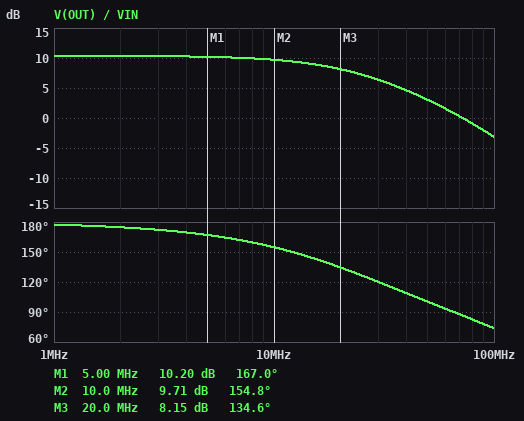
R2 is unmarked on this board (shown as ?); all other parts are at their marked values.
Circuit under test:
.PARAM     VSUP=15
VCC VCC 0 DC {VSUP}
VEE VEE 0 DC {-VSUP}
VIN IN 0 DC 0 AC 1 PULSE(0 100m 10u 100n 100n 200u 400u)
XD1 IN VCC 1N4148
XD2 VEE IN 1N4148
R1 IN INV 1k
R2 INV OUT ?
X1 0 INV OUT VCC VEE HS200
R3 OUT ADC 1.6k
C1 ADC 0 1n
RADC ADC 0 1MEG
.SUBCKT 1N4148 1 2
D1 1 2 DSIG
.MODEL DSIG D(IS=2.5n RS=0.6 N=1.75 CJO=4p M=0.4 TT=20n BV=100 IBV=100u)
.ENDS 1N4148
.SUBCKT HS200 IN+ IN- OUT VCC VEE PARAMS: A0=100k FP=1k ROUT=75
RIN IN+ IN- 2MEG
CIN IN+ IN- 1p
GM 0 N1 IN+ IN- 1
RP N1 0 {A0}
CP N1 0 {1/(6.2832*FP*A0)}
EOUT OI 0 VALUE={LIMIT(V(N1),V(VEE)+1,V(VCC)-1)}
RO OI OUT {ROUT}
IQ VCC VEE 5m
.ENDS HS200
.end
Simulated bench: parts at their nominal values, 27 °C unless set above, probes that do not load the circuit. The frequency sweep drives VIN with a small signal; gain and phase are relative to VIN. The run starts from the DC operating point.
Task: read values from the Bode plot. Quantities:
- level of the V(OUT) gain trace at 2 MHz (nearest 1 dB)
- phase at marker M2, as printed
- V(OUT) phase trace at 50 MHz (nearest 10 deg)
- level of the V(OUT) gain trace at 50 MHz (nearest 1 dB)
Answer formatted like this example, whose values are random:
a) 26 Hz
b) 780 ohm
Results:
a) 10 dB
b) 154.8 deg
c) 100 deg
d) 3 dB
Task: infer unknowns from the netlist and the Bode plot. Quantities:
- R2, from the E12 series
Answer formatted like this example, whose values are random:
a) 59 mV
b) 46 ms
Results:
a) 3.3 kΩ
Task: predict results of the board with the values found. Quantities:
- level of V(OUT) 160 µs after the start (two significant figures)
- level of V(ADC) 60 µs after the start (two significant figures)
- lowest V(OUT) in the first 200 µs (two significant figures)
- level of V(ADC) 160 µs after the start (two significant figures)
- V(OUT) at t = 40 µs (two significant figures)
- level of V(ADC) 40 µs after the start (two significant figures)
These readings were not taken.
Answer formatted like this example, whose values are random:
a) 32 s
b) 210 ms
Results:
a) -330 mV
b) -330 mV
c) -330 mV
d) -330 mV
e) -330 mV
f) -330 mV
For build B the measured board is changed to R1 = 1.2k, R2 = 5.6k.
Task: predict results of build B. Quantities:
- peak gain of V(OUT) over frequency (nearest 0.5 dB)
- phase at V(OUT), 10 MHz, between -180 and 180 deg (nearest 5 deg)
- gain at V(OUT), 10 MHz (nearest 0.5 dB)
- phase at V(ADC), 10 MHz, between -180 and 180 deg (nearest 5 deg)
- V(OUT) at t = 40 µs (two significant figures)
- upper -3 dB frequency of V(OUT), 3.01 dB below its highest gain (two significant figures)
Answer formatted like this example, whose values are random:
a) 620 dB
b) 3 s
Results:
a) 13.5 dB
b) 150 deg
c) 12.5 dB
d) 60 deg
e) -470 mV
f) 19 MHz
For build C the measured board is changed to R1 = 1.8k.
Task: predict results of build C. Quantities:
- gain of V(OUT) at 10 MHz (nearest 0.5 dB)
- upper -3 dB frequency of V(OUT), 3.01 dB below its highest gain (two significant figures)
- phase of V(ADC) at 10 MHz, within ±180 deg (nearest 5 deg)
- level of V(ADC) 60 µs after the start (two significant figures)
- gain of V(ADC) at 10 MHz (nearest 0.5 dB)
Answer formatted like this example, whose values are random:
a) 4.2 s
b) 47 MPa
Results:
a) 5.0 dB
b) 43 MHz
c) 75 deg
d) -180 mV
e) -35.0 dB
